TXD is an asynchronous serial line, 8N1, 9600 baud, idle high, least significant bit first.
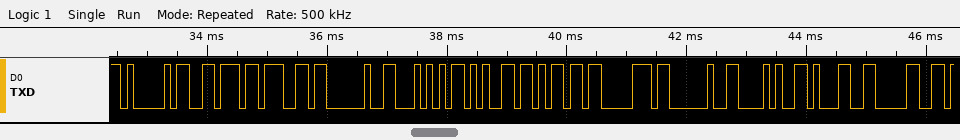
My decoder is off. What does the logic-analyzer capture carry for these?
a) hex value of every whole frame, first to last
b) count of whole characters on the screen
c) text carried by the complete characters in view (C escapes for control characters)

41 76 67 20 54 65 6D 70 20 28 31 30
12
"Avg Temp (10"
